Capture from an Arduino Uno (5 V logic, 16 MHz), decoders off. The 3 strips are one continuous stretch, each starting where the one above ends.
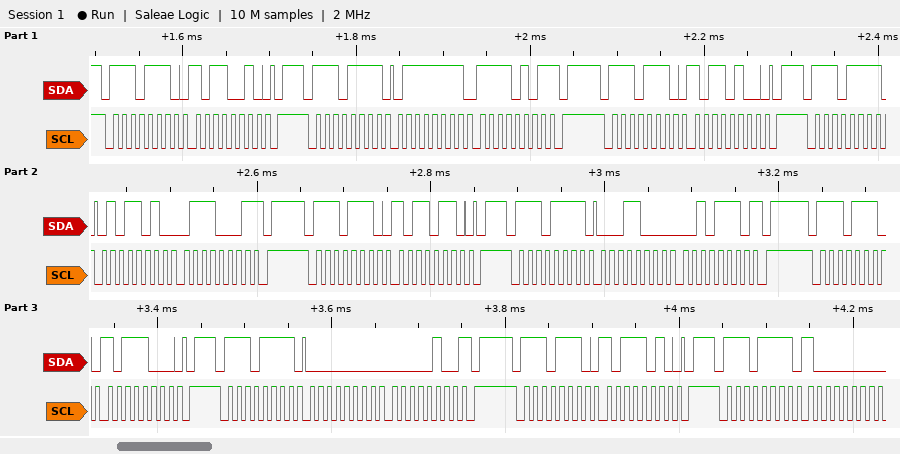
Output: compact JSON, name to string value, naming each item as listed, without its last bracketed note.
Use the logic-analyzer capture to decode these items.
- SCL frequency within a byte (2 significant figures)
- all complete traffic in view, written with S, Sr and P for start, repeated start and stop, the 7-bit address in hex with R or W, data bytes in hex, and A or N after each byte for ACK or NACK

{"SCL frequency within a byte": "100 kHz", "all complete traffic in view, written with S, Sr and P for start, repeated start and stop, the 7-bit address in hex with R or W, data bytes in hex, and A or N after each byte for ACK or NACK": "S 77W A B2 A P S 77R A 7F A F5 N P S 77W A B4 A P S 77R A 5A A 71 N P S 77W A B6 A P S 77R A 18 A 2E N P S 77W A B8 A P S 77R A 00 A 04 N P S 77W A BA A P S 77R A 80 A"}
